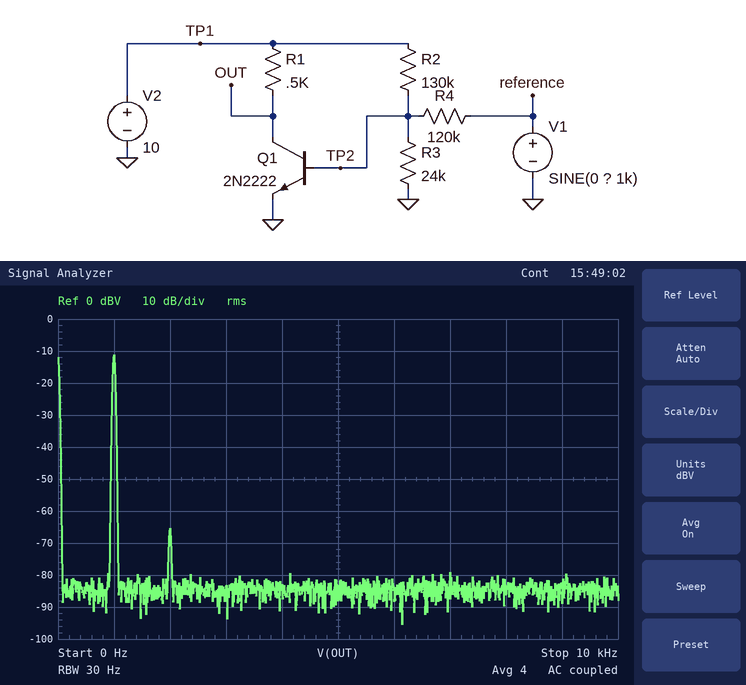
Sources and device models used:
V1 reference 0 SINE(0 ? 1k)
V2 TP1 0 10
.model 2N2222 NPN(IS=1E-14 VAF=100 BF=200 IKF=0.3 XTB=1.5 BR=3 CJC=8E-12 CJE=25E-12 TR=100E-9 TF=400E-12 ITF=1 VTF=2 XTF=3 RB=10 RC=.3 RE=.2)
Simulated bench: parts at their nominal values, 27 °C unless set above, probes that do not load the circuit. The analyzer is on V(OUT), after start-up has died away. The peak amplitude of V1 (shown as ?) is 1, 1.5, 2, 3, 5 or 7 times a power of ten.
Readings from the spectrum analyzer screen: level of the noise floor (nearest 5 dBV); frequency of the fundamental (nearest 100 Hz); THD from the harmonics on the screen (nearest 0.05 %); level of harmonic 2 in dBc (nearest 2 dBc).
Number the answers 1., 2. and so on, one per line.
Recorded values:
1. -85 dBV
2. 1.0 kHz
3. 0.20 %
4. -54 dBc
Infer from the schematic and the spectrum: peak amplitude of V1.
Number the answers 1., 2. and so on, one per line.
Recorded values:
1. 500 mV
